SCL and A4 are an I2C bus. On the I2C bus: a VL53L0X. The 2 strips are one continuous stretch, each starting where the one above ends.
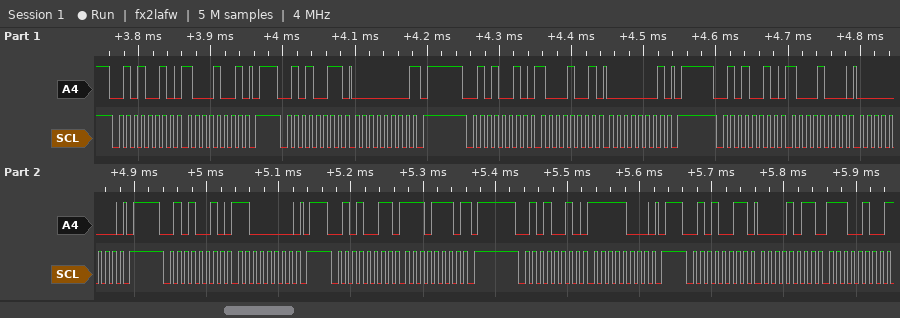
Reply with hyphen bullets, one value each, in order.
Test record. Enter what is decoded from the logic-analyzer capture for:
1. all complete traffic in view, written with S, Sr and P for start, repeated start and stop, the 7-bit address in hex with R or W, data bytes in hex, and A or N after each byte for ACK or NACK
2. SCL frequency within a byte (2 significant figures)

- S 29W A 89 A P S 29R A 00 N P S 29W A 89 A 01 A P S 29W A 88 A 00 A P S 29W A C0 A P S 29R A EE N P S 29W A F8 A P S 29R A 0B A E4 N
- 100 kHz
